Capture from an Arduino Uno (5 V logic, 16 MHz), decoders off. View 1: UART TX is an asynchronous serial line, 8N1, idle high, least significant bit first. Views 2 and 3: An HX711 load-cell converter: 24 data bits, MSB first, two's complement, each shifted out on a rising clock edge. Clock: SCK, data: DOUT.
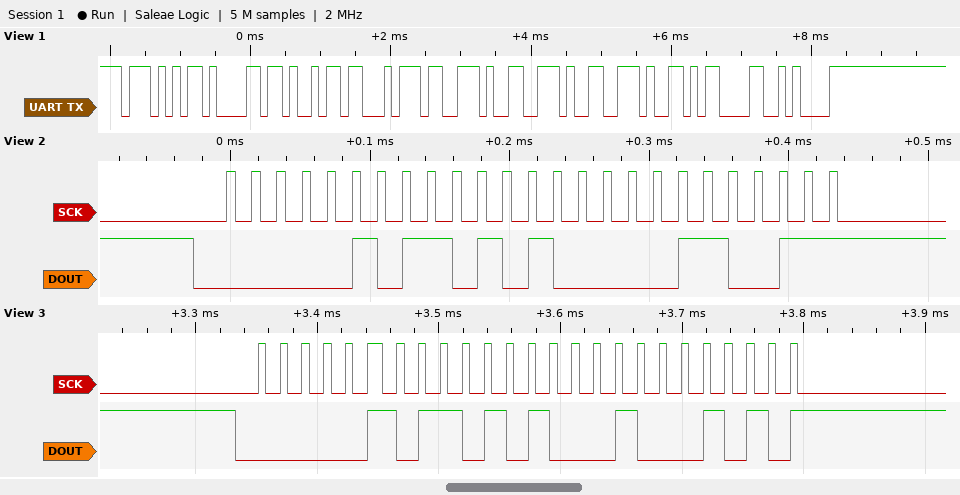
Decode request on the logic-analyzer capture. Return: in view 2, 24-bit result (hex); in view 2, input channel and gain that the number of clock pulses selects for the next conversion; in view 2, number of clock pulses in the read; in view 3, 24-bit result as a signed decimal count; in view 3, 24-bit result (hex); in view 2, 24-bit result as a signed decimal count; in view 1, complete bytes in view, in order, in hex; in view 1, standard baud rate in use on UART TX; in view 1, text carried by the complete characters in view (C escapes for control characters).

0x05A833
channel A, gain 128
25
370826
0x05A88A
370739
57 61 69 74 2E 2E 2E 0D 0A
9600 baud
"Wait...\r\n"
